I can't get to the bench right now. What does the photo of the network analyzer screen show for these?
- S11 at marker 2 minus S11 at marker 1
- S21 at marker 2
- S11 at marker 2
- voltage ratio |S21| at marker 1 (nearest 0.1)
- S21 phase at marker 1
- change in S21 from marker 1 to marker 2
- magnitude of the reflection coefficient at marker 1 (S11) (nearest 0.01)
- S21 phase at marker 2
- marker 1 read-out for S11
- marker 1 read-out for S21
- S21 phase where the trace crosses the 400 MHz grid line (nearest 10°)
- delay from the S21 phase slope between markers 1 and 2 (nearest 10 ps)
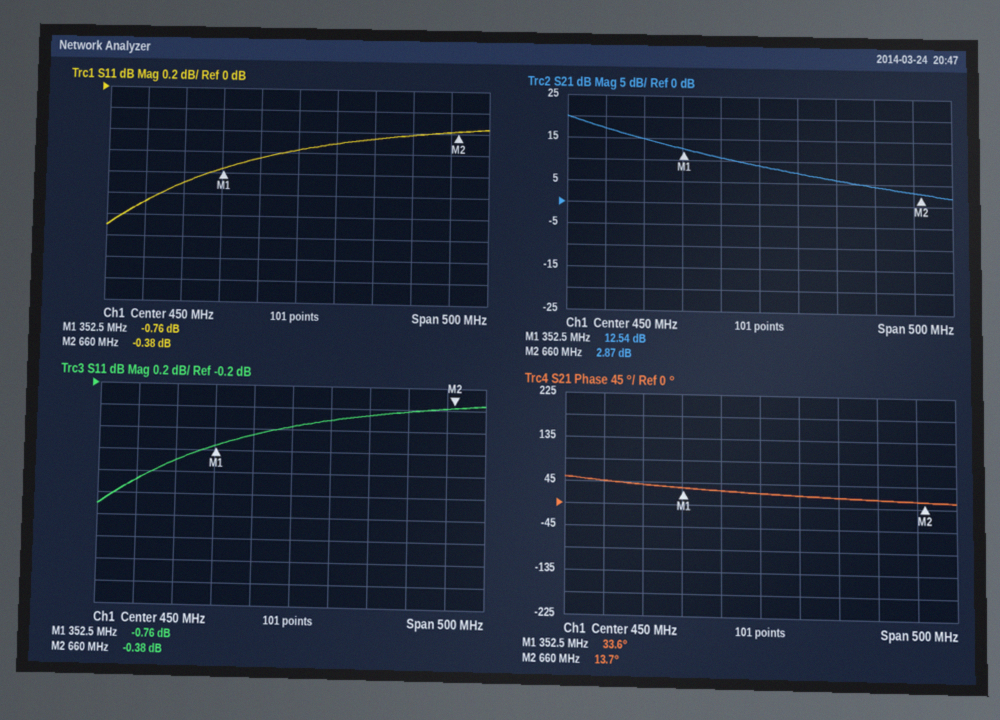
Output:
0.38 dB
2.87 dB
-0.38 dB
4.2
33.6°
-9.67 dB
0.92
13.7°
-0.76 dB
12.54 dB
30°
180 ps
